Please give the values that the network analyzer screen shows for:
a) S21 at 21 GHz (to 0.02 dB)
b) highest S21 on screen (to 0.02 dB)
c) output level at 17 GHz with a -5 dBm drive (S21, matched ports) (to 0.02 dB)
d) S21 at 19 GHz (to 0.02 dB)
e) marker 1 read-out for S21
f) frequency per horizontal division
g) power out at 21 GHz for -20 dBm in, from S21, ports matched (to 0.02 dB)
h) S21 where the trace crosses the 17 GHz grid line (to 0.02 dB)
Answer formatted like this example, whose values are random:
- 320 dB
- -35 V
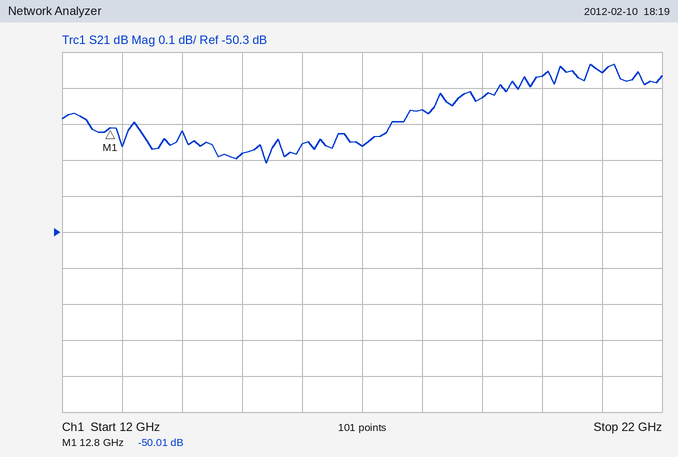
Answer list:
- -49.86 dB
- -49.84 dB
- -55.06 dBm
- -49.92 dB
- -50.01 dB
- 1 GHz
- -69.86 dBm
- -50.06 dB
